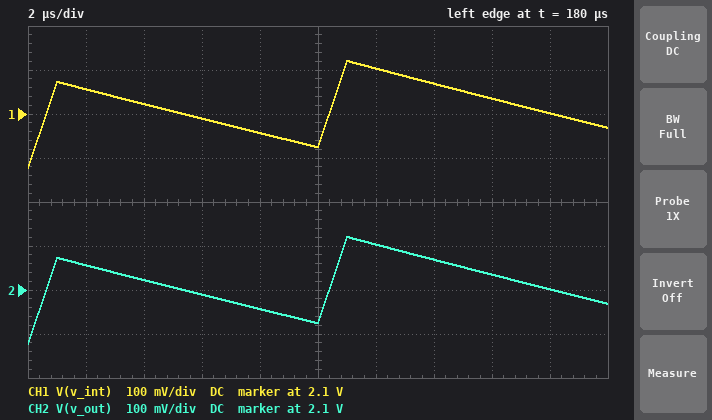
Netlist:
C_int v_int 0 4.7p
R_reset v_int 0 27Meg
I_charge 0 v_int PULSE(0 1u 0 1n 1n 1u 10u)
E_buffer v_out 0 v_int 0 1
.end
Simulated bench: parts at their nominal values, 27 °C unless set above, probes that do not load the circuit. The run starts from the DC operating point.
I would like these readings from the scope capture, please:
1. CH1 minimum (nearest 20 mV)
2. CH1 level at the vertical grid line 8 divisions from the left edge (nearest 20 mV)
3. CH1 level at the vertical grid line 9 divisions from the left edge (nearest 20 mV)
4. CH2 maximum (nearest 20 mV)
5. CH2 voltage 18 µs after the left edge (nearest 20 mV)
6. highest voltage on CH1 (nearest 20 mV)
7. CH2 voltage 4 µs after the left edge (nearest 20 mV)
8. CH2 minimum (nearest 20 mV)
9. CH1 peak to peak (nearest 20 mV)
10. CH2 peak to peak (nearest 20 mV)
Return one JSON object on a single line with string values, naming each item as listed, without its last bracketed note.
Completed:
{"CH1 minimum": "1.98 V", "CH1 level at the vertical grid line 8 divisions from the left edge": "2.14 V", "CH1 level at the vertical grid line 9 divisions from the left edge": "2.10 V", "CH2 maximum": "2.22 V", "CH2 voltage 18 µs after the left edge": "2.10 V", "highest voltage on CH1": "2.22 V", "CH2 voltage 4 µs after the left edge": "2.12 V", "CH2 minimum": "1.98 V", "CH1 peak to peak": "240 mV", "CH2 peak to peak": "240 mV"}
